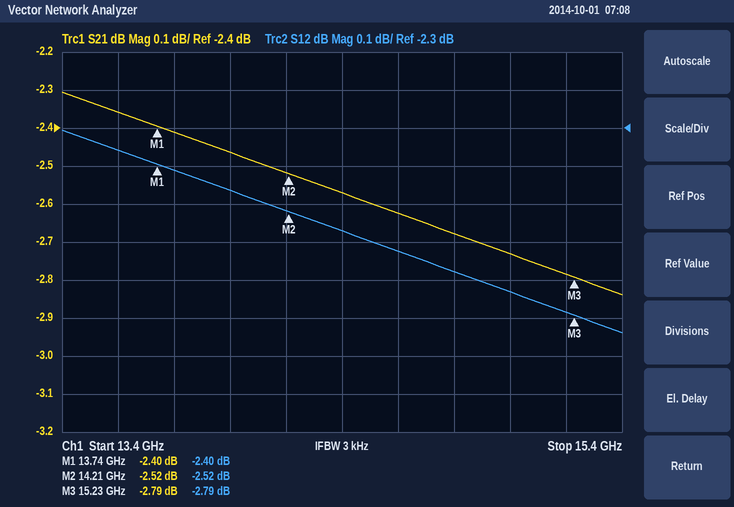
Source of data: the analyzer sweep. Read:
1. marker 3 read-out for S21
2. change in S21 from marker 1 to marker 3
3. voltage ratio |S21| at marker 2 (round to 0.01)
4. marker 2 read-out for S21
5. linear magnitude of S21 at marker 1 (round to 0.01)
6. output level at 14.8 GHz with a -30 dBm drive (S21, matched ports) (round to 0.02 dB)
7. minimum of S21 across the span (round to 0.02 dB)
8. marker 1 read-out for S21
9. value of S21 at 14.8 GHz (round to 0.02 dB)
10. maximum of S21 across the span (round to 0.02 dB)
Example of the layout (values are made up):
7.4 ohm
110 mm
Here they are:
-2.79 dB
-0.39 dB
0.75
-2.52 dB
0.76
-32.68 dBm
-2.84 dB
-2.40 dB
-2.68 dB
-2.30 dB
